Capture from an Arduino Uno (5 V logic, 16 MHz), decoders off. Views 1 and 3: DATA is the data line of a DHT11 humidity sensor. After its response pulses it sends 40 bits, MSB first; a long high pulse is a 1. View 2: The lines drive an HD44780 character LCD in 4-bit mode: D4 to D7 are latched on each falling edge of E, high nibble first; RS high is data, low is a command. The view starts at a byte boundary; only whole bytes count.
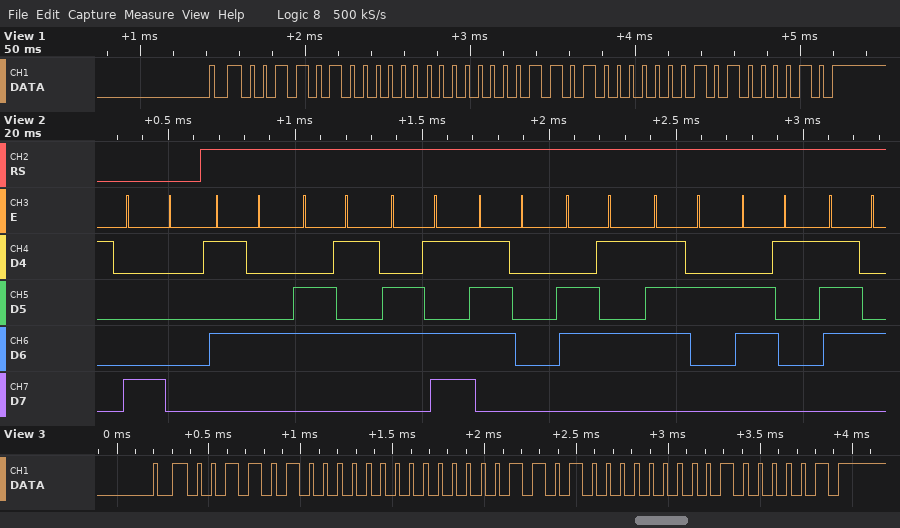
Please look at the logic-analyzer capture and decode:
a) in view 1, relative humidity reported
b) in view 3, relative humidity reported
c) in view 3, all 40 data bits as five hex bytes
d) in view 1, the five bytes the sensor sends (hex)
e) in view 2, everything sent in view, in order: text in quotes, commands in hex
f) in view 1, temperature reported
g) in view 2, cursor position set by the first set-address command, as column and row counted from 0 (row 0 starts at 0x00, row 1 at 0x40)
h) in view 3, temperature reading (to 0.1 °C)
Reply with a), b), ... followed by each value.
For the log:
a) 52 %
b) 52 %
c) 34 00 0D 00 41
d) 34 00 0D 01 42
e) 0x80 "Temperat"
f) 13.1 °C
g) column 0, row 0
h) 13.0 °C
